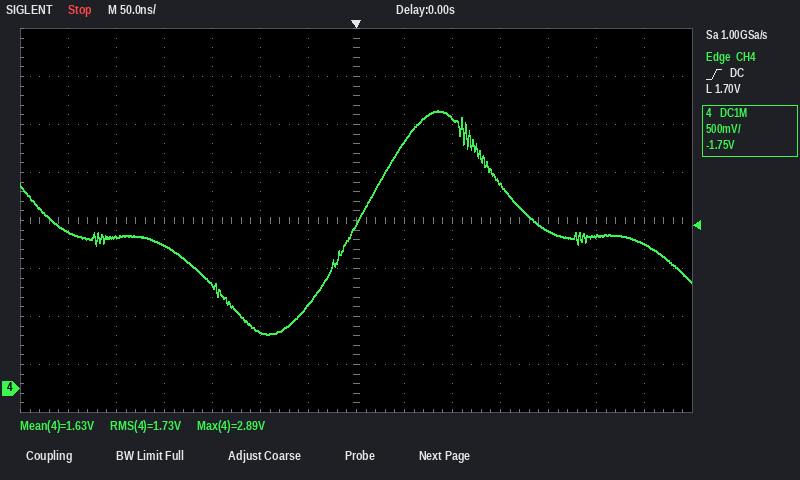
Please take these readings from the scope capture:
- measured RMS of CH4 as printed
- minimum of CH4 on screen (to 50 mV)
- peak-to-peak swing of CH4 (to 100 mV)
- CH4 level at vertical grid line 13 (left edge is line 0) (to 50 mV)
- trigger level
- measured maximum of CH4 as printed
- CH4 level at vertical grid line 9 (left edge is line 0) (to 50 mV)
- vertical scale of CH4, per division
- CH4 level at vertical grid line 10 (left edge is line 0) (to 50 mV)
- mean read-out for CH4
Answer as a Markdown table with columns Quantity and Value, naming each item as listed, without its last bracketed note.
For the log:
| Quantity | Value |
|---|---|
| measured RMS of CH4 as printed | 1.73 V |
| minimum of CH4 on screen | 550 mV |
| peak-to-peak swing of CH4 | 2.30 V |
| CH4 level at vertical grid line 13 (left edge is line 0) | 1.50 V |
| trigger level | 1.70 V |
| measured maximum of CH4 as printed | 2.89 V |
| CH4 level at vertical grid line 9 (left edge is line 0) | 2.80 V |
| vertical scale of CH4, per division | 500 mV |
| CH4 level at vertical grid line 10 (left edge is line 0) | 2.15 V |
| mean read-out for CH4 | 1.63 V |
